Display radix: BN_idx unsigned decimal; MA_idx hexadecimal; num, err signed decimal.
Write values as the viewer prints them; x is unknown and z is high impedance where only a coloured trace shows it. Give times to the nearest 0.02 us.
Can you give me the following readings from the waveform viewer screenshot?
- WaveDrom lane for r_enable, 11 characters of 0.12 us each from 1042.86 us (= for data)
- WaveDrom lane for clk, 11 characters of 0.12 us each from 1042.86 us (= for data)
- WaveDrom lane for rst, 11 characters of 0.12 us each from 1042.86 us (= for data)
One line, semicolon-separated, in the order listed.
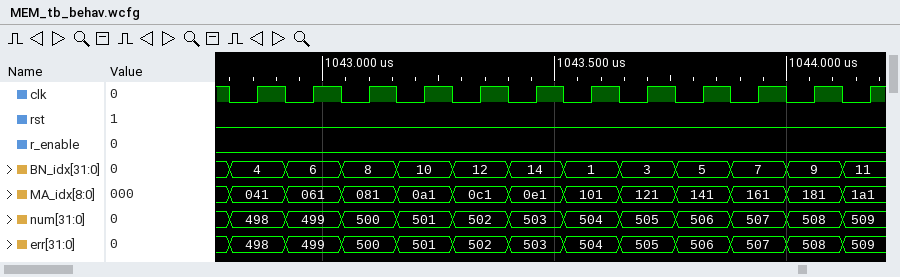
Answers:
{name: 'r_enable', wave: '0..........'}; {name: 'clk', wave: 'p..........'}; {name: 'rst', wave: '0..........'}
